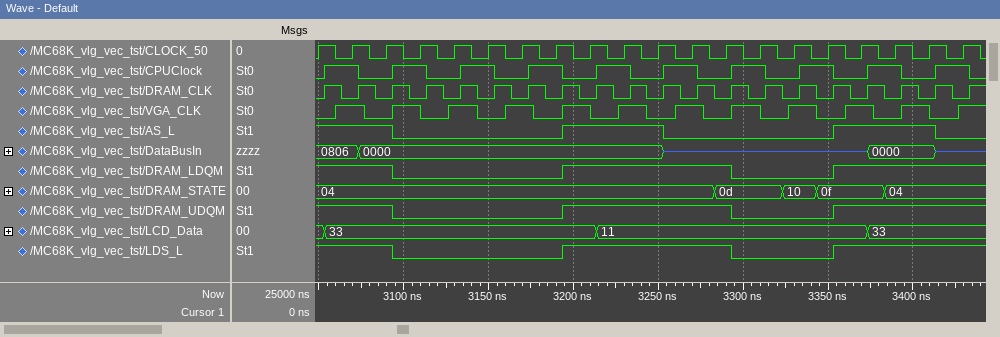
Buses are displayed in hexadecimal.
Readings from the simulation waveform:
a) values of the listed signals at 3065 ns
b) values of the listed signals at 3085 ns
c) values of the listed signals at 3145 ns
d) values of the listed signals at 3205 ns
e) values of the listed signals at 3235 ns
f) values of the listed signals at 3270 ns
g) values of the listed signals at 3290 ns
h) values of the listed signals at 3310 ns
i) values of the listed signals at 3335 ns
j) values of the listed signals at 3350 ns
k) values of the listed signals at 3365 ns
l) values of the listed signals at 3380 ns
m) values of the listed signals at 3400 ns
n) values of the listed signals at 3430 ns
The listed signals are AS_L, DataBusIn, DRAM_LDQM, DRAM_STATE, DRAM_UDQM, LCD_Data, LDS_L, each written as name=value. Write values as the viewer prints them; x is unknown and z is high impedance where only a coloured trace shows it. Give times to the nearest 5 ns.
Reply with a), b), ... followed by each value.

a) AS_L=1, DataBusIn=0806, DRAM_LDQM=1, DRAM_STATE=04, DRAM_UDQM=1, LCD_Data=33, LDS_L=1
b) AS_L=1, DataBusIn=0000, DRAM_LDQM=1, DRAM_STATE=04, DRAM_UDQM=1, LCD_Data=33, LDS_L=1
c) AS_L=0, DataBusIn=0000, DRAM_LDQM=0, DRAM_STATE=04, DRAM_UDQM=0, LCD_Data=33, LDS_L=0
d) AS_L=1, DataBusIn=0000, DRAM_LDQM=1, DRAM_STATE=04, DRAM_UDQM=1, LCD_Data=33, LDS_L=1
e) AS_L=1, DataBusIn=0000, DRAM_LDQM=1, DRAM_STATE=04, DRAM_UDQM=1, LCD_Data=11, LDS_L=1
f) AS_L=0, DataBusIn=z, DRAM_LDQM=1, DRAM_STATE=04, DRAM_UDQM=1, LCD_Data=11, LDS_L=1
g) AS_L=0, DataBusIn=z, DRAM_LDQM=1, DRAM_STATE=0d, DRAM_UDQM=1, LCD_Data=11, LDS_L=1
h) AS_L=0, DataBusIn=z, DRAM_LDQM=0, DRAM_STATE=0d, DRAM_UDQM=0, LCD_Data=11, LDS_L=0
i) AS_L=0, DataBusIn=z, DRAM_LDQM=0, DRAM_STATE=10, DRAM_UDQM=0, LCD_Data=11, LDS_L=0
j) AS_L=0, DataBusIn=z, DRAM_LDQM=0, DRAM_STATE=0f, DRAM_UDQM=0, LCD_Data=11, LDS_L=0
k) AS_L=1, DataBusIn=z, DRAM_LDQM=1, DRAM_STATE=0f, DRAM_UDQM=1, LCD_Data=11, LDS_L=1
l) AS_L=1, DataBusIn=0000, DRAM_LDQM=1, DRAM_STATE=0f, DRAM_UDQM=1, LCD_Data=33, LDS_L=1
m) AS_L=1, DataBusIn=0000, DRAM_LDQM=1, DRAM_STATE=04, DRAM_UDQM=1, LCD_Data=33, LDS_L=1
n) AS_L=0, DataBusIn=z, DRAM_LDQM=1, DRAM_STATE=04, DRAM_UDQM=1, LCD_Data=33, LDS_L=1
